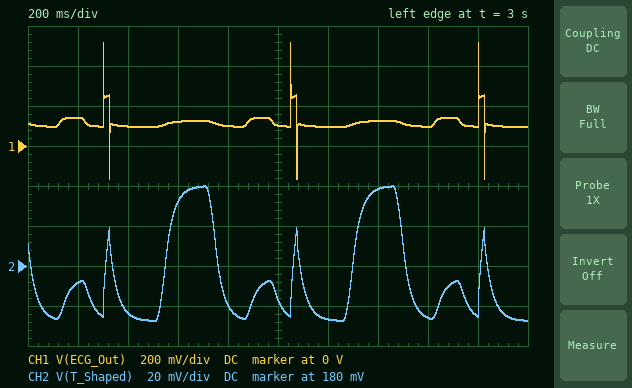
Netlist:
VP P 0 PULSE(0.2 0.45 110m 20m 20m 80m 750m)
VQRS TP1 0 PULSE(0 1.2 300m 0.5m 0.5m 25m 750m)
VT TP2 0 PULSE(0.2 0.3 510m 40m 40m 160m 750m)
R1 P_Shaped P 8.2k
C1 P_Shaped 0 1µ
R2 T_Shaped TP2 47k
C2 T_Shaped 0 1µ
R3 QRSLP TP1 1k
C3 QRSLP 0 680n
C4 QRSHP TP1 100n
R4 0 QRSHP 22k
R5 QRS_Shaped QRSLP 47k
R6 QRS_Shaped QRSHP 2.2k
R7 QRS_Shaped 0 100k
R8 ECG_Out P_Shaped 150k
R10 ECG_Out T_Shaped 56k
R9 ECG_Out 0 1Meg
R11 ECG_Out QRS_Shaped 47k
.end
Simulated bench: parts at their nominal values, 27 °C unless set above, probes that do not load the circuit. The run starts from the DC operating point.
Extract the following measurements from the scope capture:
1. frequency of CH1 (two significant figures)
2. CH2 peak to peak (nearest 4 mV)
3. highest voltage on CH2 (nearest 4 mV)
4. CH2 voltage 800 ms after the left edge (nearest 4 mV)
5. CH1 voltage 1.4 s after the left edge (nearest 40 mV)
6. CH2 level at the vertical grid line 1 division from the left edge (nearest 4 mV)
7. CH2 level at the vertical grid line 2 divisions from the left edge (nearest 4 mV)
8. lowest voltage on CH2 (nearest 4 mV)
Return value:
1.3 Hz
68 mV
220 mV
160 mV
120 mV
172 mV
156 mV
152 mV
